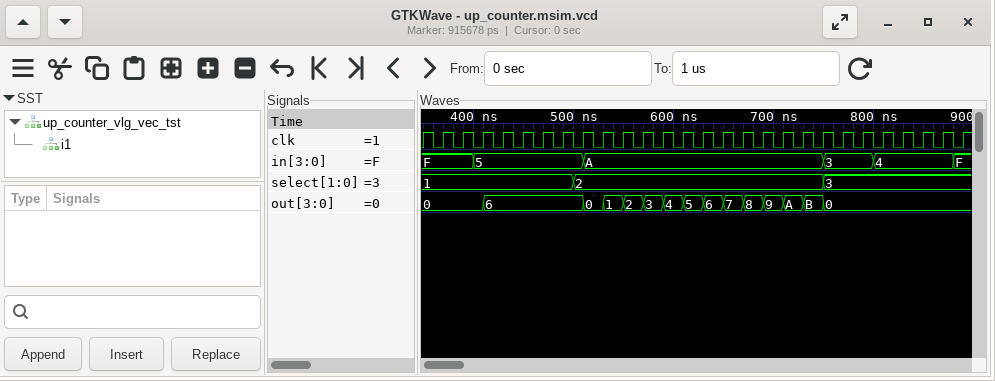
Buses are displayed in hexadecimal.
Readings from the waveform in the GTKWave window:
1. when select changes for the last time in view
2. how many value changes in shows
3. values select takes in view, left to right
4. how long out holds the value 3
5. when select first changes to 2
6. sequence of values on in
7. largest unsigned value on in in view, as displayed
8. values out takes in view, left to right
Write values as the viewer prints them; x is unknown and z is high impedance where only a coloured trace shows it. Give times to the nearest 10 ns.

750 ns
5
1, 2, 3
20 ns
500 ns
F, 5, A, 3, 4, F
F
0, 6, 0, 1, 2, 3, 4, 5, 6, 7, 8, 9, A, B, 0
